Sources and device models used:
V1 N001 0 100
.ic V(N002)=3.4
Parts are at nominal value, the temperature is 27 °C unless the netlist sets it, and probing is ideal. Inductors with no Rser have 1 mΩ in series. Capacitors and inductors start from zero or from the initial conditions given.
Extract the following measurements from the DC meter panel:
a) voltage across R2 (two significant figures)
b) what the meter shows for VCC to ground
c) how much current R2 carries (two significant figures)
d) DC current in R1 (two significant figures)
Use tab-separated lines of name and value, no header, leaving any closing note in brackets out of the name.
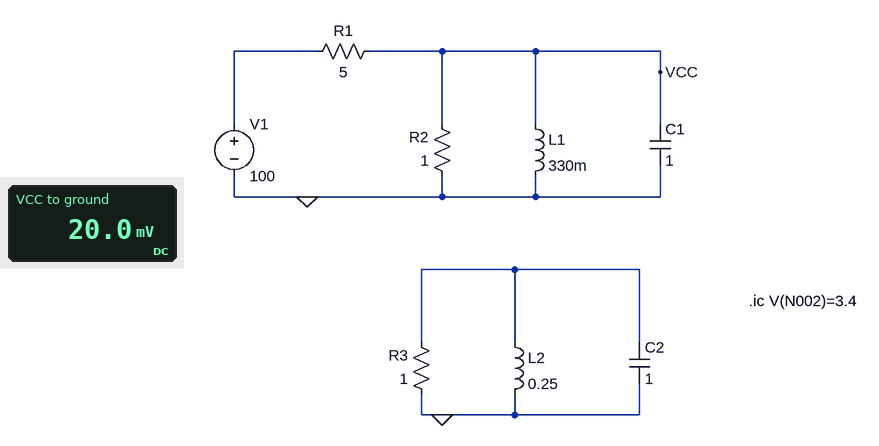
voltage across R2	20 mV
what the meter shows for VCC to ground	20.0 mV
how much current R2 carries	20 mA
DC current in R1	20 A
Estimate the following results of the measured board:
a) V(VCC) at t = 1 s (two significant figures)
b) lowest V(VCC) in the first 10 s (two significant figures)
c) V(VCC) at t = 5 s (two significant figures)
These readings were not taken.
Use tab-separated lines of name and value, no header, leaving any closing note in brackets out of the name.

V(VCC) at t = 1 s	6.7 V
lowest V(VCC) in the first 10 s	-2.3 V
V(VCC) at t = 5 s	590 mV
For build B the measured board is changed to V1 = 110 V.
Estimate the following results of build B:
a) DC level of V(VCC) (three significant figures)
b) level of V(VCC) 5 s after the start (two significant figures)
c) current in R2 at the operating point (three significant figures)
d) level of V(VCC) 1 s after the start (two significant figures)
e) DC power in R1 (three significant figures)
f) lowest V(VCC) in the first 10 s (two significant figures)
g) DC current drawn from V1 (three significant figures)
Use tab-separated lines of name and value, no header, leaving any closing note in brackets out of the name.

DC level of V(VCC)	22.0 mV
level of V(VCC) 5 s after the start	650 mV
current in R2 at the operating point	22.0 mA
level of V(VCC) 1 s after the start	7.4 V
DC power in R1	2.42 kW
lowest V(VCC) in the first 10 s	-2.5 V
DC current drawn from V1	22.0 A
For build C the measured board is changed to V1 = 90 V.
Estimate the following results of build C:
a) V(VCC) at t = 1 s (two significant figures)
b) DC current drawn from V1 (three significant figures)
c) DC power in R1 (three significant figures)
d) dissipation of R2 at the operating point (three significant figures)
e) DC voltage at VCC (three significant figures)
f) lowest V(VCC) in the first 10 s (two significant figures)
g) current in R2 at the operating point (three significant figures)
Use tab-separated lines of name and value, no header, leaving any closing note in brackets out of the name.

V(VCC) at t = 1 s	6.0 V
DC current drawn from V1	18.0 A
DC power in R1	1.62 kW
dissipation of R2 at the operating point	323 µW
DC voltage at VCC	18.0 mV
lowest V(VCC) in the first 10 s	-2.1 V
current in R2 at the operating point	18.0 mA
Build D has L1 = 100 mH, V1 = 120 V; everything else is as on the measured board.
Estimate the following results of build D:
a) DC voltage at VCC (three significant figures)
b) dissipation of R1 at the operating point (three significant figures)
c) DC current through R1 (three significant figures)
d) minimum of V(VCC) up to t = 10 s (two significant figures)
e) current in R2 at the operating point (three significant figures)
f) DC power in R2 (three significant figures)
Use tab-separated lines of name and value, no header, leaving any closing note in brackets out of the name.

DC voltage at VCC	24.0 mV
dissipation of R1 at the operating point	2.88 kW
DC current through R1	24.0 A
minimum of V(VCC) up to t = 10 s	-3.1 V
current in R2 at the operating point	24.0 mA
DC power in R2	575 µW
